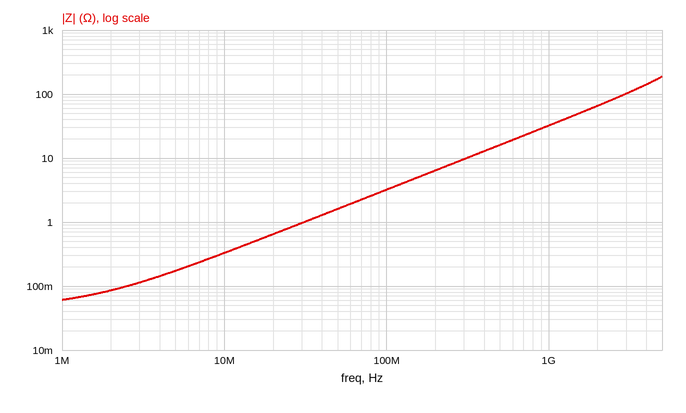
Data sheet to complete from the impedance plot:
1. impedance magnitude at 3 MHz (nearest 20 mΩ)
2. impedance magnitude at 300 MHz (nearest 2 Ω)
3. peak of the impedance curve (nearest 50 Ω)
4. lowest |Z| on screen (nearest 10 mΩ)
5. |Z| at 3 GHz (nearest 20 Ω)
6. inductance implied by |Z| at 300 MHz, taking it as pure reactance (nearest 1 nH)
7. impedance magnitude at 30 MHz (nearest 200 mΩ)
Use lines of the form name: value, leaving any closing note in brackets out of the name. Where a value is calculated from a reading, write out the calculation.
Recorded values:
impedance magnitude at 3 MHz: 120 mΩ
impedance magnitude at 300 MHz: 10 Ω
peak of the impedance curve: 200 Ω
lowest |Z| on screen: 60 mΩ
|Z| at 3 GHz: 100 Ω
inductance implied by |Z| at 300 MHz, taking it as pure reactance: L = 10 Ω/(2π × 300 MHz) ≈ 5 nH
impedance magnitude at 30 MHz: 1.0 Ω
